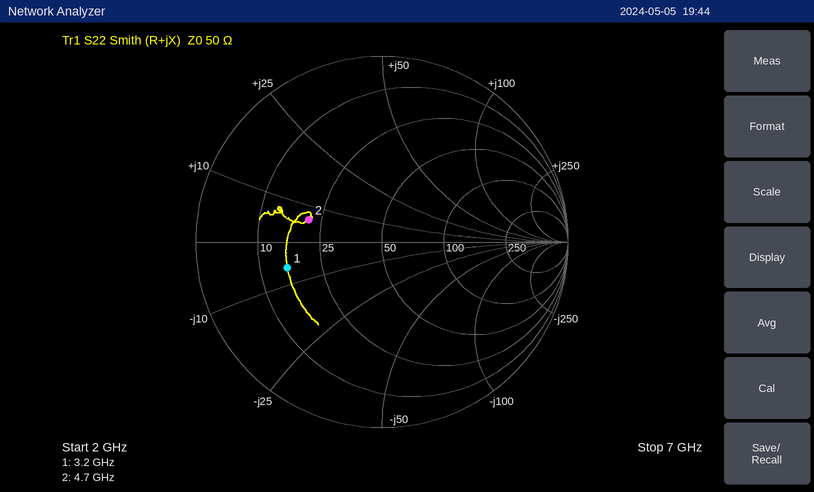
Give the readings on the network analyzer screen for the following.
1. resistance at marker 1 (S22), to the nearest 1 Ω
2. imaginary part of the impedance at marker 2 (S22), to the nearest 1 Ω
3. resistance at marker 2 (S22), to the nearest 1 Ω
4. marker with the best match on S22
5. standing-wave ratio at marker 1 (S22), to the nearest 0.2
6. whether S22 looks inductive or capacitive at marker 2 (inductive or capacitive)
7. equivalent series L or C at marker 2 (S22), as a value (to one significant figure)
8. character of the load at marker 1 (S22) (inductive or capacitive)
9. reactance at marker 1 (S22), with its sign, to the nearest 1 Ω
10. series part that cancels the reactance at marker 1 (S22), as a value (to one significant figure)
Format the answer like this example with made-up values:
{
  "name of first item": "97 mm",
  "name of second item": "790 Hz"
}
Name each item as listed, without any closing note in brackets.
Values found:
{
  "resistance at marker 1 (S22), to the nearest 1 Ω": "16 Ω",
  "imaginary part of the impedance at marker 2 (S22), to the nearest 1 Ω": "+6 Ω",
  "resistance at marker 2 (S22), to the nearest 1 Ω": "21 Ω",
  "marker with the best match on S22": "marker 2",
  "standing-wave ratio at marker 1 (S22), to the nearest 0.2": "3.2",
  "whether S22 looks inductive or capacitive at marker 2": "inductive",
  "equivalent series L or C at marker 2 (S22), as a value": "200 pH",
  "character of the load at marker 1 (S22)": "capacitive",
  "reactance at marker 1 (S22), with its sign, to the nearest 1 Ω": "-6 Ω",
  "series part that cancels the reactance at marker 1 (S22), as a value": "300 pH"
}
